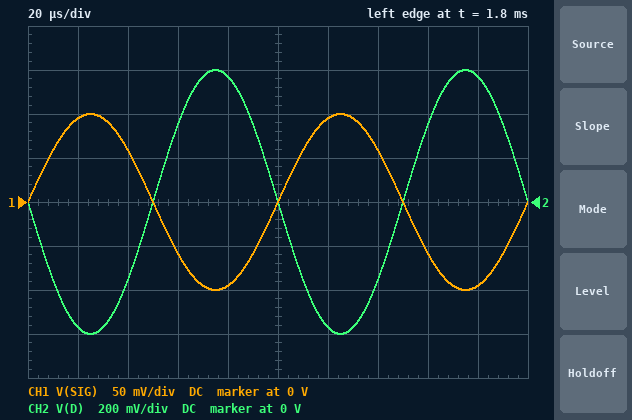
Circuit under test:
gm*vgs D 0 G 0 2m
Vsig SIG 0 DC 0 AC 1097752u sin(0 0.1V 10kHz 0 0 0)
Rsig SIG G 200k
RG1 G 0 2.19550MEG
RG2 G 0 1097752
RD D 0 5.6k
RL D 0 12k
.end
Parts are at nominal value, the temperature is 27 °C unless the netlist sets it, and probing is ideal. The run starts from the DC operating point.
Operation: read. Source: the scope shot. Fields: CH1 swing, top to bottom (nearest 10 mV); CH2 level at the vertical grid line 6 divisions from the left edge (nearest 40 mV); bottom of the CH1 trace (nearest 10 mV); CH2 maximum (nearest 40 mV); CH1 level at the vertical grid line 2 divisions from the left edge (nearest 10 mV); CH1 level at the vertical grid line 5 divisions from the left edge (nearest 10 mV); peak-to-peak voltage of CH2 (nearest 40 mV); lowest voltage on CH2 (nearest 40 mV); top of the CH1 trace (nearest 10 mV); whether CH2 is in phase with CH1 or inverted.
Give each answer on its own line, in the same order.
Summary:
200 mV
-560 mV
-100 mV
600 mV
60 mV
0 V
1.20 V
-600 mV
100 mV
inverted
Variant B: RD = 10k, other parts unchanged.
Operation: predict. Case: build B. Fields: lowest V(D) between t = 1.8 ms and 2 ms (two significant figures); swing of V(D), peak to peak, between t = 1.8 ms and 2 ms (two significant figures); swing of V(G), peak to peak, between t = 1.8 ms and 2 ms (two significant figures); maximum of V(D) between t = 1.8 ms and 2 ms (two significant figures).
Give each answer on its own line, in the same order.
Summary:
-860 mV
1.7 V
160 mV
860 mV
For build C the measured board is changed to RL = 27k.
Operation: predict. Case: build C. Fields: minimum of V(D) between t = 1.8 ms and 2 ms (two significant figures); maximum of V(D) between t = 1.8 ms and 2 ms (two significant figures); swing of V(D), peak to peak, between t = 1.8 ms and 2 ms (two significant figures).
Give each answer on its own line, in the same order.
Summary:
-730 mV
730 mV
1.5 V
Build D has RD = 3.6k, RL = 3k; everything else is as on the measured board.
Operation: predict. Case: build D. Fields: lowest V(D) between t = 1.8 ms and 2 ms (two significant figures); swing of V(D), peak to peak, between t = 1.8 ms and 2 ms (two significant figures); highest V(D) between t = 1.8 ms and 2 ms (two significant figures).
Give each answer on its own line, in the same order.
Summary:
-260 mV
510 mV
260 mV
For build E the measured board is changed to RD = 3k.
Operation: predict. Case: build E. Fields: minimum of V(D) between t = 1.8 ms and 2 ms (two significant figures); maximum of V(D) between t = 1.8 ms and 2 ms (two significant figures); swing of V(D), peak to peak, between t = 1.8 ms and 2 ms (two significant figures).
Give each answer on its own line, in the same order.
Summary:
-380 mV
380 mV
750 mV
